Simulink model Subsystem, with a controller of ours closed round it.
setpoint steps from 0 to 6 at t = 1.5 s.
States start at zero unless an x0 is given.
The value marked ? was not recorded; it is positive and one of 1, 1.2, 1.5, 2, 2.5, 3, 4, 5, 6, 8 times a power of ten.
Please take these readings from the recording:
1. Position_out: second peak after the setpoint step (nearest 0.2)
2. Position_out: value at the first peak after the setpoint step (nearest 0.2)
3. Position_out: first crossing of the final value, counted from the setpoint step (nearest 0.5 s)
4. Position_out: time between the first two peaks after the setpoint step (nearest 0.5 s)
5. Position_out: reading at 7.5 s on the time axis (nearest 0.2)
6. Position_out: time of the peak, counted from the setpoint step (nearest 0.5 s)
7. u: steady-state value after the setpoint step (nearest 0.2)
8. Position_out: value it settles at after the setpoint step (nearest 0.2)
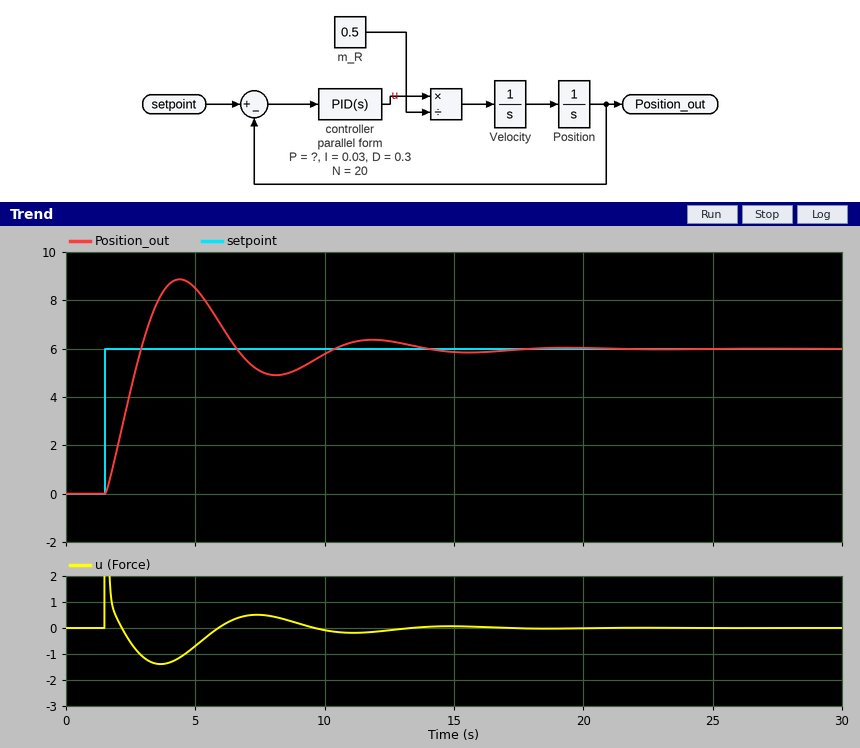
6.4
8.8
1.5 s
7.5 s
5.0
3.0 s
0.0
6.0
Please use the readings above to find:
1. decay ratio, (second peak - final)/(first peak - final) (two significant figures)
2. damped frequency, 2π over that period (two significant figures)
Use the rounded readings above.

0.14
0.84 rad/s
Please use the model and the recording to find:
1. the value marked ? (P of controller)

0.4
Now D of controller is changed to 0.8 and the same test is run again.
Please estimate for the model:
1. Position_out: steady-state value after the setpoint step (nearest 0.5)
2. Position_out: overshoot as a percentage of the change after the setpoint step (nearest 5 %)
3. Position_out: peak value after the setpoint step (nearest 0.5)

6.0
20 %
7.0
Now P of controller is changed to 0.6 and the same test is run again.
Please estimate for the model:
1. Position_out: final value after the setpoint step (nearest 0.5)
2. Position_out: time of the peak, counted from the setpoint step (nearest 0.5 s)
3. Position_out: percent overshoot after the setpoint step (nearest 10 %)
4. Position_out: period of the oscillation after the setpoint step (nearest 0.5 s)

6.0
2.5 s
50 %
6.0 s
